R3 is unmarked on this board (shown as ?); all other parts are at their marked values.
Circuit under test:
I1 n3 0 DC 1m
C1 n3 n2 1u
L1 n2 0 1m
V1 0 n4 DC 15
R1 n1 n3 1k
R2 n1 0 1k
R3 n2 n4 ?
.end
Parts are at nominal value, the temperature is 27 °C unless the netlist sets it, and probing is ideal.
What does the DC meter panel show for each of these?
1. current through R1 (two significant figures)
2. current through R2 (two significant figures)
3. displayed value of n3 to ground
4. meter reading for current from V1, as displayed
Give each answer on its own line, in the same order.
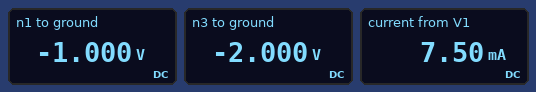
1.0 mA
1.0 mA
-2.000 V
7.50 mA
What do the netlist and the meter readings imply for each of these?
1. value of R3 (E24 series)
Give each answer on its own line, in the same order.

2 kΩ
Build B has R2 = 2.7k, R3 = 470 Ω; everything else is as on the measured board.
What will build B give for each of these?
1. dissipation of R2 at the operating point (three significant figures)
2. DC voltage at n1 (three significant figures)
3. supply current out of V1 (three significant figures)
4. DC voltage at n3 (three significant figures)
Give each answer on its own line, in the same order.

2.70 mW
-2.70 V
31.9 mA
-3.70 V
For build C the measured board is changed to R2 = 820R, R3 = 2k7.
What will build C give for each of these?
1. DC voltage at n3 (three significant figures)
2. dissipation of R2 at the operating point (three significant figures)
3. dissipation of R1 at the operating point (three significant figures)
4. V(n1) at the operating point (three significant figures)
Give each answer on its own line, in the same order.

-1.82 V
820 µW
1.00 mW
-820 mV
